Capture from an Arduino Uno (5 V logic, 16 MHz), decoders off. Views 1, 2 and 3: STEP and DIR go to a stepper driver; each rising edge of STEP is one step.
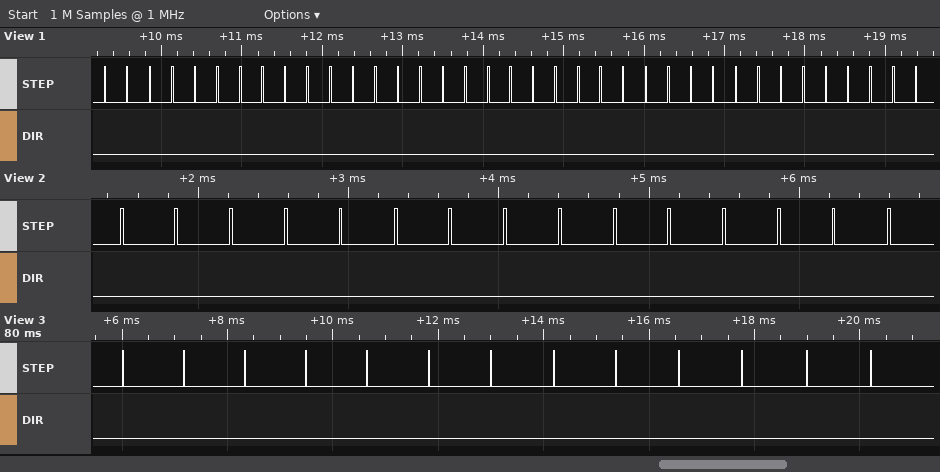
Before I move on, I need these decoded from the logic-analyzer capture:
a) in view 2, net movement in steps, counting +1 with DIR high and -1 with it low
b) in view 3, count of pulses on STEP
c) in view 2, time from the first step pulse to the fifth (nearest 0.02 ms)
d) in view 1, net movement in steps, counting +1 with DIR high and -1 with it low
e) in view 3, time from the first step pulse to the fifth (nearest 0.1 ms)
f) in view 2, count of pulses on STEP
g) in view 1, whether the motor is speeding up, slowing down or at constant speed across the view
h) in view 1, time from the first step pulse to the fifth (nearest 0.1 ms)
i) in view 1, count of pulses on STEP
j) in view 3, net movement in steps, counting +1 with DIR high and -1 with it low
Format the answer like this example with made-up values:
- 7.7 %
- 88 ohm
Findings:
- -15
- 13
- 1.46 ms
- -37
- 4.6 ms
- 15
- constant speed
- 1.1 ms
- 37
- -13
